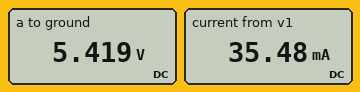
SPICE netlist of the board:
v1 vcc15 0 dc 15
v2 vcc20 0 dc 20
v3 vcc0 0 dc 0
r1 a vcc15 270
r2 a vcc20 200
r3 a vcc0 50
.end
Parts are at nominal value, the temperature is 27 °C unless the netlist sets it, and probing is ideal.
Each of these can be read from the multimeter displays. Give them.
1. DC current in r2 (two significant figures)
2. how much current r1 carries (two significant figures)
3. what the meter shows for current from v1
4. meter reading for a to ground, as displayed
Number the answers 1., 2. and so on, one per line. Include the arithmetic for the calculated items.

1. (20 V - 5.419 V) / 200 Ω = 73 mA
2. (15 V - 5.419 V) / 270 Ω = 35 mA
3. 35.48 mA
4. 5.419 V
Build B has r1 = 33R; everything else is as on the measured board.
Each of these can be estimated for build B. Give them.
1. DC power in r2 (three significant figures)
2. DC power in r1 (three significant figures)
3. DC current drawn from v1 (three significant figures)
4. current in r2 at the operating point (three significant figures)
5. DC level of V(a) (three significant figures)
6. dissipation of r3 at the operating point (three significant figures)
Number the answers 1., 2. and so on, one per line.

1. 497 mW
2. 749 mW
3. 151 mA
4. 49.9 mA
5. 10.0 V
6. 2.01 W
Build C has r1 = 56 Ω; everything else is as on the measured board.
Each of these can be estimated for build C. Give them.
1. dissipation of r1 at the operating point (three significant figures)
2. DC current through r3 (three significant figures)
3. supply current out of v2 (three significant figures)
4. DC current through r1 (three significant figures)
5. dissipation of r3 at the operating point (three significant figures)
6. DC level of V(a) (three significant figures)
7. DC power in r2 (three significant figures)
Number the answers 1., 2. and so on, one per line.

1. 735 mW
2. 172 mA
3. 57.1 mA
4. 115 mA
5. 1.47 W
6. 8.58 V
7. 652 mW
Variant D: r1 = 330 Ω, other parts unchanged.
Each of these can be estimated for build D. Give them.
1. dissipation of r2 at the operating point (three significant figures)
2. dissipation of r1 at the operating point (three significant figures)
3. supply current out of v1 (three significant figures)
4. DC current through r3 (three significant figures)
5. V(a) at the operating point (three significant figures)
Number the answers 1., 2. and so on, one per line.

1. 1.10 W
2. 292 mW
3. 29.7 mA
4. 104 mA
5. 5.19 V
